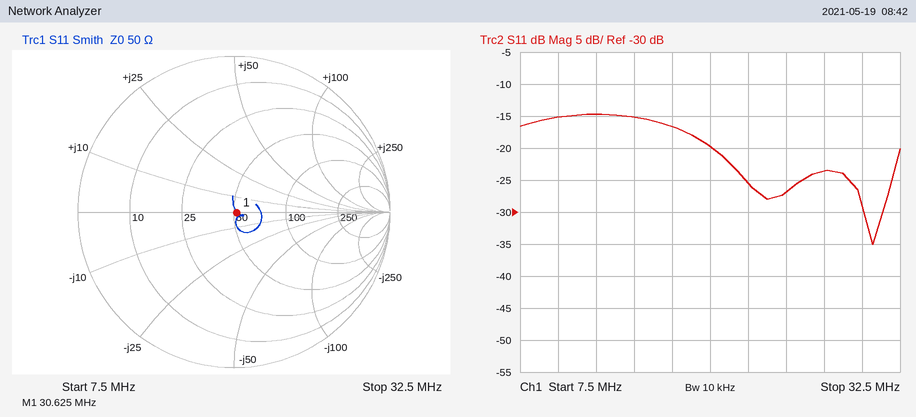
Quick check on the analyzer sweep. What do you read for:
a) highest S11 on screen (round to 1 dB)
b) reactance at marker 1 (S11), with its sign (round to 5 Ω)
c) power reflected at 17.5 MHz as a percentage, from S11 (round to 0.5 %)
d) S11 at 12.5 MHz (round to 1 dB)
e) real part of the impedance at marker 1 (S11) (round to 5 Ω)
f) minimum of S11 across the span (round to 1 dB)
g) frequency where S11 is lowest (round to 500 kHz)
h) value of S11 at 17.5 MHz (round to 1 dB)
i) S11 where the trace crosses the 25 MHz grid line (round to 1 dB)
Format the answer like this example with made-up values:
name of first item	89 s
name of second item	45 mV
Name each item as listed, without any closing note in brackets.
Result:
highest S11 on screen	-15 dB
reactance at marker 1 (S11), with its sign	0 Ω
power reflected at 17.5 MHz as a percentage, from S11	2.0 %
S11 at 12.5 MHz	-15 dB
real part of the impedance at marker 1 (S11)	50 Ω
minimum of S11 across the span	-35 dB
frequency where S11 is lowest	30.5 MHz
value of S11 at 17.5 MHz	-17 dB
S11 where the trace crosses the 25 MHz grid line	-27 dB
